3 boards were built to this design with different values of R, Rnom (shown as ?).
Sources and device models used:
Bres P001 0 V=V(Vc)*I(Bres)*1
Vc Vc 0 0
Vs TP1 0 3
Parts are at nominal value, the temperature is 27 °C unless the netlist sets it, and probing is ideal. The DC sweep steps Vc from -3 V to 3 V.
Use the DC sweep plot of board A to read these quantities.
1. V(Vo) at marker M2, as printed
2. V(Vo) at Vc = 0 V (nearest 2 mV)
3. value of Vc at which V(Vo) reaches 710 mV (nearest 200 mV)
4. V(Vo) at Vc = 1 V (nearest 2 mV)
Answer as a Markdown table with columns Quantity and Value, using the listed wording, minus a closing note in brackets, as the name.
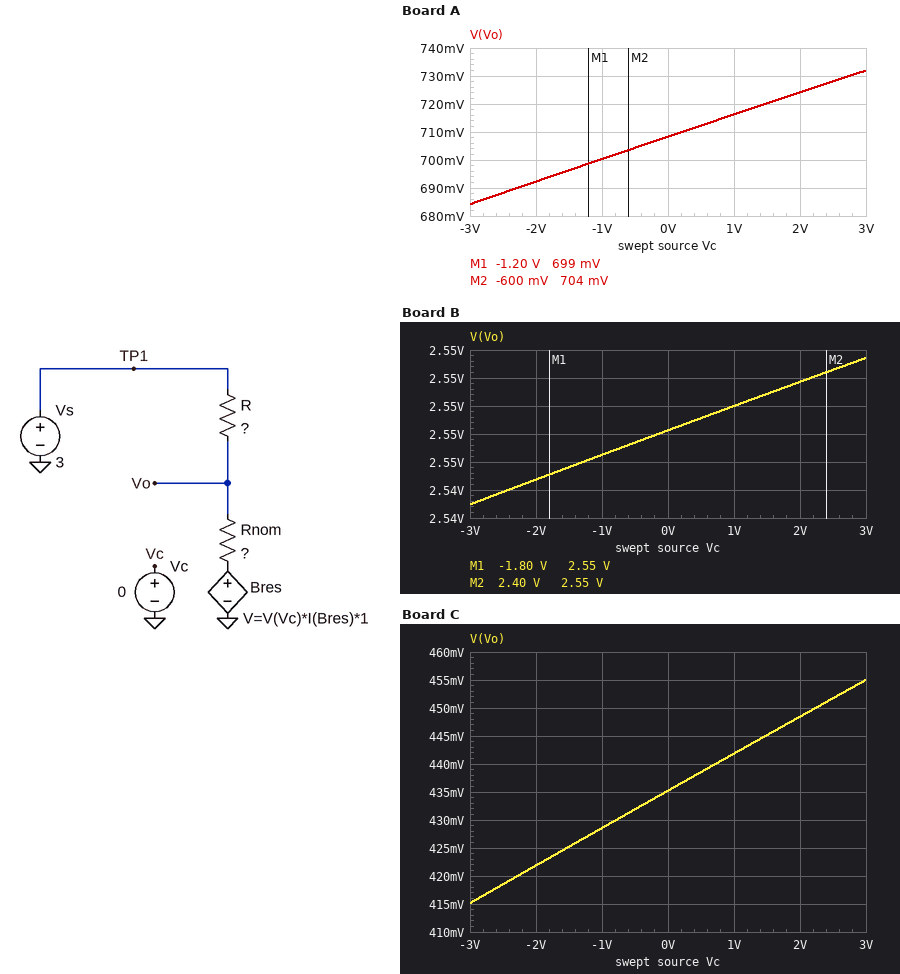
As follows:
| Quantity | Value |
|---|---|
| V(Vo) at marker M2, as printed | 704 mV |
| V(Vo) at Vc = 0 V | 708 mV |
| value of Vc at which V(Vo) reaches 710 mV | 200 mV |
| V(Vo) at Vc = 1 V | 716 mV |
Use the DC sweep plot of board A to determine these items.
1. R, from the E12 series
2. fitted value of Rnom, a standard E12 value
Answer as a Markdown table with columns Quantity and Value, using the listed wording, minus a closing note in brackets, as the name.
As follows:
| Quantity | Value |
|---|---|
| R, from the E12 series | 220 Ω |
| fitted value of Rnom, a standard E12 value | 68 Ω |
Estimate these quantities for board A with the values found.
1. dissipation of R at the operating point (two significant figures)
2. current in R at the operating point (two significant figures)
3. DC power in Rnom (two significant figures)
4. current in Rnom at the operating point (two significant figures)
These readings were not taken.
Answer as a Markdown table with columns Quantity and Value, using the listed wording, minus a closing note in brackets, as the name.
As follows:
| Quantity | Value |
|---|---|
| dissipation of R at the operating point | 24 mW |
| current in R at the operating point | 10 mA |
| DC power in Rnom | 7.4 mW |
| current in Rnom at the operating point | 10 mA |
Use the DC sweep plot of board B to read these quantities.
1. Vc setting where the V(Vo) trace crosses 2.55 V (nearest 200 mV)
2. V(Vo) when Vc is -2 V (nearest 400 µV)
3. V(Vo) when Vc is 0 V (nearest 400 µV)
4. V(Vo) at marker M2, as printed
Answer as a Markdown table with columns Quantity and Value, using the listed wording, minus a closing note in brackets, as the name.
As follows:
| Quantity | Value |
|---|---|
| Vc setting where the V(Vo) trace crosses 2.55 V | 1.0 V |
| V(Vo) when Vc is -2 V | 2.5448 V |
| V(Vo) when Vc is 0 V | 2.5484 V |
| V(Vo) at marker M2, as printed | 2.55 V |
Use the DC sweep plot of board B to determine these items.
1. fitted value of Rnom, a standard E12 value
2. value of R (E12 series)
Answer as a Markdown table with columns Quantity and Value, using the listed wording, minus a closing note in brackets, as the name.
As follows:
| Quantity | Value |
|---|---|
| fitted value of Rnom, a standard E12 value | 220 Ω |
| value of R | 39 Ω |
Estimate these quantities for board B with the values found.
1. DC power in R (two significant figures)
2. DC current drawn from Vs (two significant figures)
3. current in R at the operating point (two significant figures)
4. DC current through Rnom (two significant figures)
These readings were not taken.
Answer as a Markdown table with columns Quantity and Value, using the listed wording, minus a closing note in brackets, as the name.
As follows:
| Quantity | Value |
|---|---|
| DC power in R | 5.2 mW |
| DC current drawn from Vs | 12 mA |
| current in R at the operating point | 12 mA |
| DC current through Rnom | 12 mA |
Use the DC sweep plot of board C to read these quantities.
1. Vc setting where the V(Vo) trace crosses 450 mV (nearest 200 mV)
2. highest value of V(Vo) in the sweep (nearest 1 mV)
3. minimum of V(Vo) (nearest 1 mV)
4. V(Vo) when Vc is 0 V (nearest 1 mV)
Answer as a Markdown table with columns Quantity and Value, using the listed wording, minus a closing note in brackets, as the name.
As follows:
| Quantity | Value |
|---|---|
| Vc setting where the V(Vo) trace crosses 450 mV | 2.2 V |
| highest value of V(Vo) in the sweep | 455 mV |
| minimum of V(Vo) | 415 mV |
| V(Vo) when Vc is 0 V | 435 mV |
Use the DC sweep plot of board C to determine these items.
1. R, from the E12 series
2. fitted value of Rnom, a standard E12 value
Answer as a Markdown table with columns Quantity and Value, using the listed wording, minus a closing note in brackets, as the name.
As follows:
| Quantity | Value |
|---|---|
| R, from the E12 series | 330 Ω |
| fitted value of Rnom, a standard E12 value | 56 Ω |
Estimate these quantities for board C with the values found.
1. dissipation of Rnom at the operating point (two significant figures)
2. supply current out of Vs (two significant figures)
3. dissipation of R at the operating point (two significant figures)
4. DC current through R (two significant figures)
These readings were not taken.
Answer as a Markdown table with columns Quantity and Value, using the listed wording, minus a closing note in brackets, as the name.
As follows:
| Quantity | Value |
|---|---|
| dissipation of Rnom at the operating point | 3.4 mW |
| supply current out of Vs | 7.8 mA |
| dissipation of R at the operating point | 20 mW |
| DC current through R | 7.8 mA |
